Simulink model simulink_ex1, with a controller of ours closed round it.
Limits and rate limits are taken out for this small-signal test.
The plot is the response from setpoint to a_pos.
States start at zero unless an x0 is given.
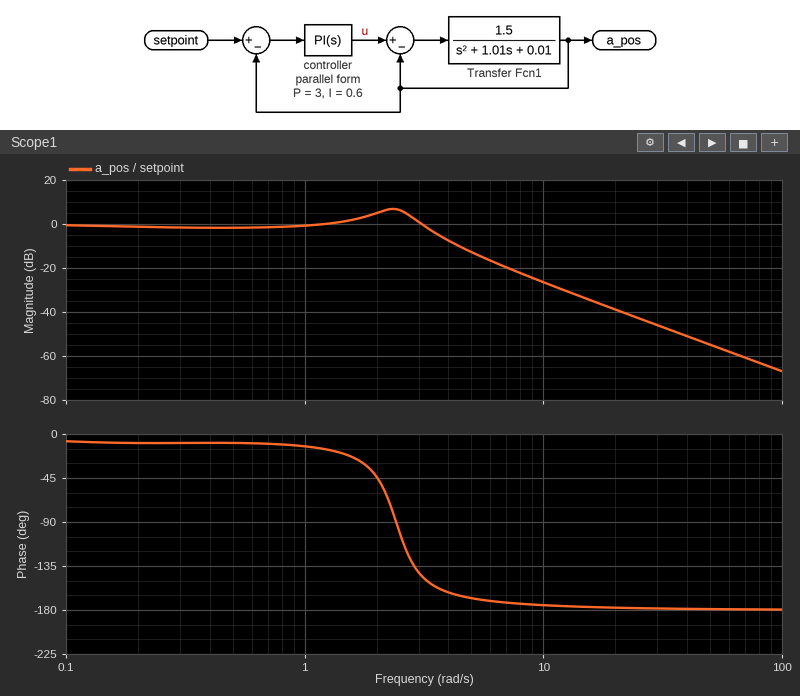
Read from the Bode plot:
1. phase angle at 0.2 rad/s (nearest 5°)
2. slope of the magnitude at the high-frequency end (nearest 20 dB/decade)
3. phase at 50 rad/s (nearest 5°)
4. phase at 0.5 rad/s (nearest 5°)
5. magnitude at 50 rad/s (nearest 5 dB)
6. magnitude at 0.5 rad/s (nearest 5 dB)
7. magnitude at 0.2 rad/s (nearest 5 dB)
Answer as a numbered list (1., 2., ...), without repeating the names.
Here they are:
1. -10°
2. -40 dB/decade
3. -180°
4. -10°
5. -55 dB
6. 0 dB
7. 0 dB
